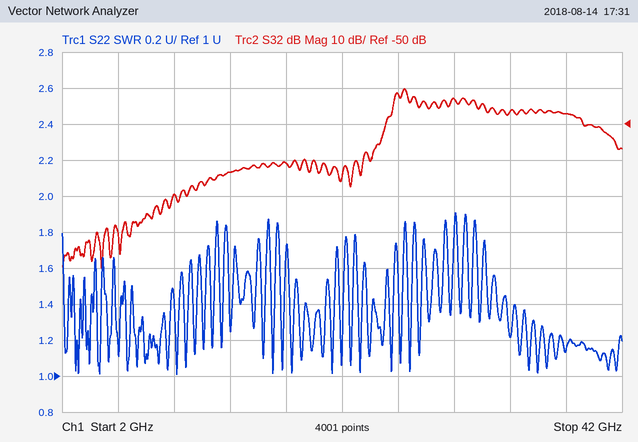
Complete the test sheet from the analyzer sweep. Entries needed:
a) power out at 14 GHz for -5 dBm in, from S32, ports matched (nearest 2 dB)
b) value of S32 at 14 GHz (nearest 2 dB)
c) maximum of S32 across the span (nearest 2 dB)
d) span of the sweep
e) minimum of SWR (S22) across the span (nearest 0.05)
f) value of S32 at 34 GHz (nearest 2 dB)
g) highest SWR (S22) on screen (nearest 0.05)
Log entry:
-68 dBm
-64 dB
-40 dB
40 GHz
1.00
-46 dB
1.90
